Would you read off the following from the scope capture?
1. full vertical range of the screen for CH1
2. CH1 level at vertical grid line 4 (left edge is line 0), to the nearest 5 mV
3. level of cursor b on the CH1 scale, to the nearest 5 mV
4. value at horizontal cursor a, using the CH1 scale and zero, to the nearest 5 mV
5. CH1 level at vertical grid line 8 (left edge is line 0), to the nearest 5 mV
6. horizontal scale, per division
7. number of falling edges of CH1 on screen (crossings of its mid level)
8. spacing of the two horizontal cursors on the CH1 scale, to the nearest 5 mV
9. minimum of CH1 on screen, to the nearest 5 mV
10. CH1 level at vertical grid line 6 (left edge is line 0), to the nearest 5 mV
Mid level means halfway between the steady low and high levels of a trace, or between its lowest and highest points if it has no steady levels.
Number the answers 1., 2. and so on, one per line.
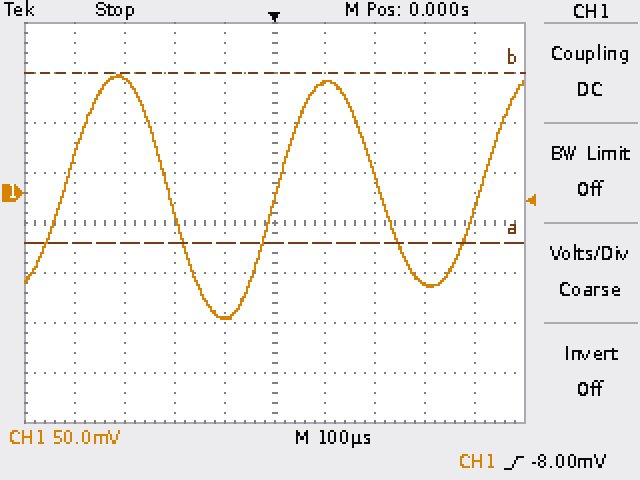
1. 400 mV
2. -125 mV
3. 120 mV
4. -50 mV
5. -90 mV
6. 100 µs
7. 2
8. 170 mV
9. -125 mV
10. 110 mV
